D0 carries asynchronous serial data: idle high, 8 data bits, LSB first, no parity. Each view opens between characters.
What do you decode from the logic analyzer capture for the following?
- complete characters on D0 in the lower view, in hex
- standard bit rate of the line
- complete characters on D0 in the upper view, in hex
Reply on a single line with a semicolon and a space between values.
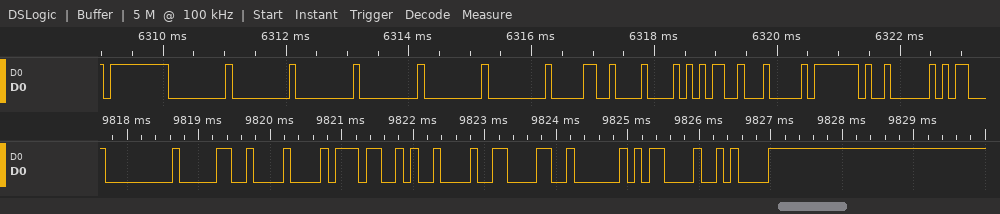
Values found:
00, 30, 08, 37, 09, 86, 02, 0D, 0A; 9600 baud; FF, 00, 00, 00, 00, 00, 00, 30, 08, 35, 04, 7F, 02
